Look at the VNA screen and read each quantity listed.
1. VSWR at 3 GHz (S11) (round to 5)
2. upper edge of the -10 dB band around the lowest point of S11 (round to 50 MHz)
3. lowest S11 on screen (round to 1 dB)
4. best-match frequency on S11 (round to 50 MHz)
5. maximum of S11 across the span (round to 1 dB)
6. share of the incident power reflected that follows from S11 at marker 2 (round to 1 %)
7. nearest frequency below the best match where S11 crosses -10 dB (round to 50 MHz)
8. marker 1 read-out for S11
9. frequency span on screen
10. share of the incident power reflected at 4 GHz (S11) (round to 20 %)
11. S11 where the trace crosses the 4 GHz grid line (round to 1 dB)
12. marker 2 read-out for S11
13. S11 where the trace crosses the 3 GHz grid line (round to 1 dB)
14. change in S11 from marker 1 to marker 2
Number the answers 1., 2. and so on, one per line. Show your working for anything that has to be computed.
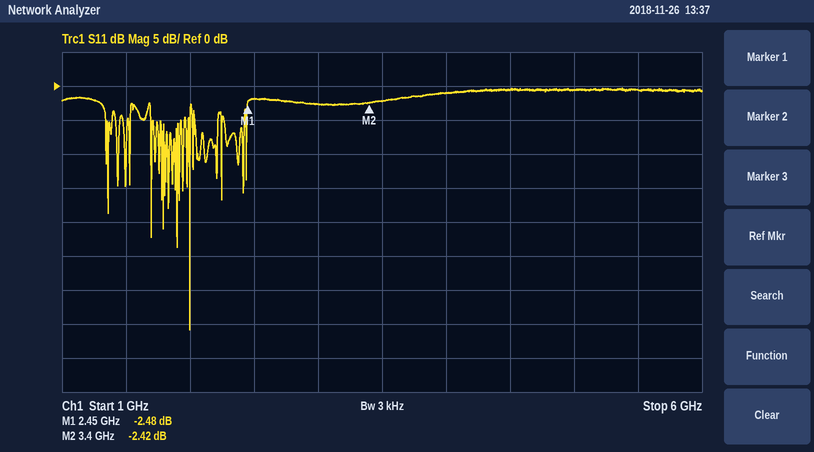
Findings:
1. |Γ| = 10^(-3/20) = 0.7079; VSWR = (1 + 0.7079)/(1 − 0.7079) ≈ 5.85, so 5 to the nearest 5
2. 2.00 GHz
3. -36 dB
4. 2.00 GHz
5. 0 dB
6. 10^(-2.42/10) ≈ 57 %
7. 2.00 GHz
8. -2.48 dB
9. 5 GHz
10. 10^(-1/10) ≈ 79.4 %, so 80 % to the nearest 20 %
11. -1 dB
12. -2.42 dB
13. -3 dB
14. -2.42 − (-2.48) = 0.06 dB
